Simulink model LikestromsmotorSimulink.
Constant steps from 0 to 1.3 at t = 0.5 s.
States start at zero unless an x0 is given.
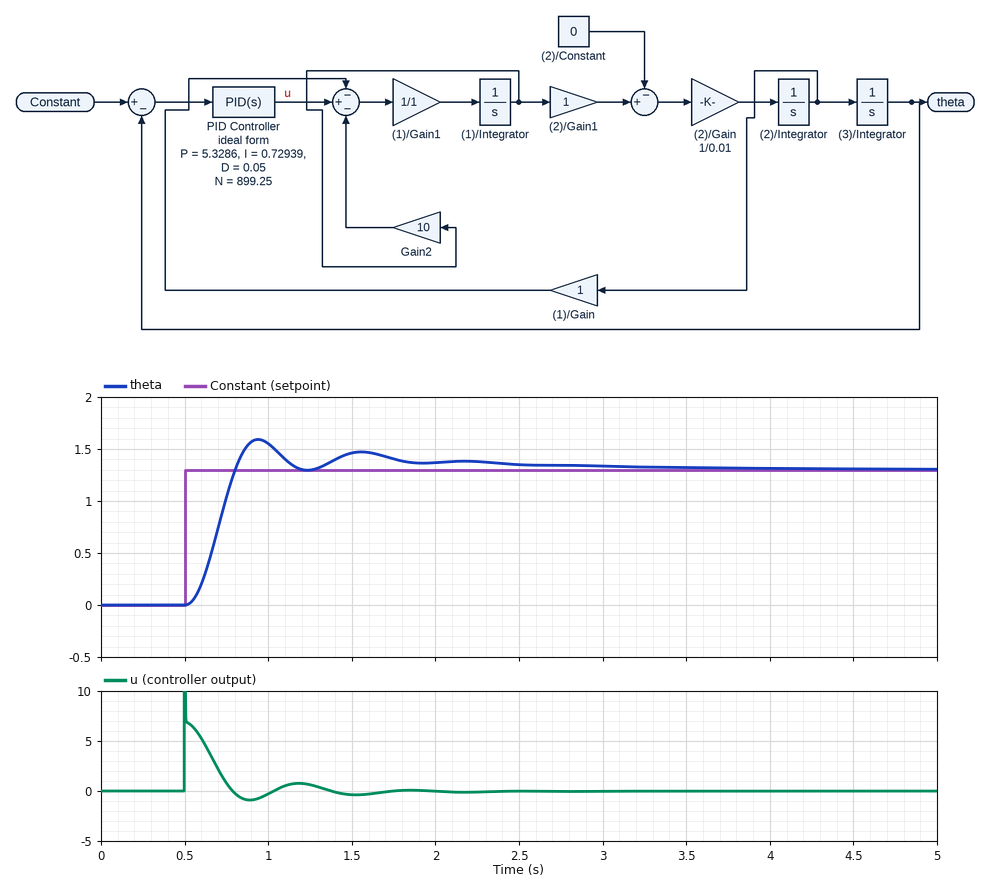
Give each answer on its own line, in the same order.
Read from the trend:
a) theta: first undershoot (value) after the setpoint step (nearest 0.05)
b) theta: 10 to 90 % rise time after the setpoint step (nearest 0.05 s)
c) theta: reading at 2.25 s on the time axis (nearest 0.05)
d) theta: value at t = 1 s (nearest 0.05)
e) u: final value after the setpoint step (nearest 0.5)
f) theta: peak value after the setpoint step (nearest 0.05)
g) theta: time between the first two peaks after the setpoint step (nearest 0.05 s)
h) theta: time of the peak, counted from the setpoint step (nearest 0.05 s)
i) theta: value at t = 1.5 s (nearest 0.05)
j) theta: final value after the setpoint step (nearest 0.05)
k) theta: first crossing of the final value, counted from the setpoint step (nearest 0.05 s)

1.30
0.20 s
1.40
1.55
0.0
1.60
0.60 s
0.45 s
1.45
1.30
0.30 s
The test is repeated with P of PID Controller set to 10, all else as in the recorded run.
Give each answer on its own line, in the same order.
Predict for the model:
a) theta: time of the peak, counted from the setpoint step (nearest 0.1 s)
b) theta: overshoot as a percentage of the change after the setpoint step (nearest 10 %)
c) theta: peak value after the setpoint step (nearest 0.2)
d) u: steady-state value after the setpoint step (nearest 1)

0.3 s
50 %
2.0
0
